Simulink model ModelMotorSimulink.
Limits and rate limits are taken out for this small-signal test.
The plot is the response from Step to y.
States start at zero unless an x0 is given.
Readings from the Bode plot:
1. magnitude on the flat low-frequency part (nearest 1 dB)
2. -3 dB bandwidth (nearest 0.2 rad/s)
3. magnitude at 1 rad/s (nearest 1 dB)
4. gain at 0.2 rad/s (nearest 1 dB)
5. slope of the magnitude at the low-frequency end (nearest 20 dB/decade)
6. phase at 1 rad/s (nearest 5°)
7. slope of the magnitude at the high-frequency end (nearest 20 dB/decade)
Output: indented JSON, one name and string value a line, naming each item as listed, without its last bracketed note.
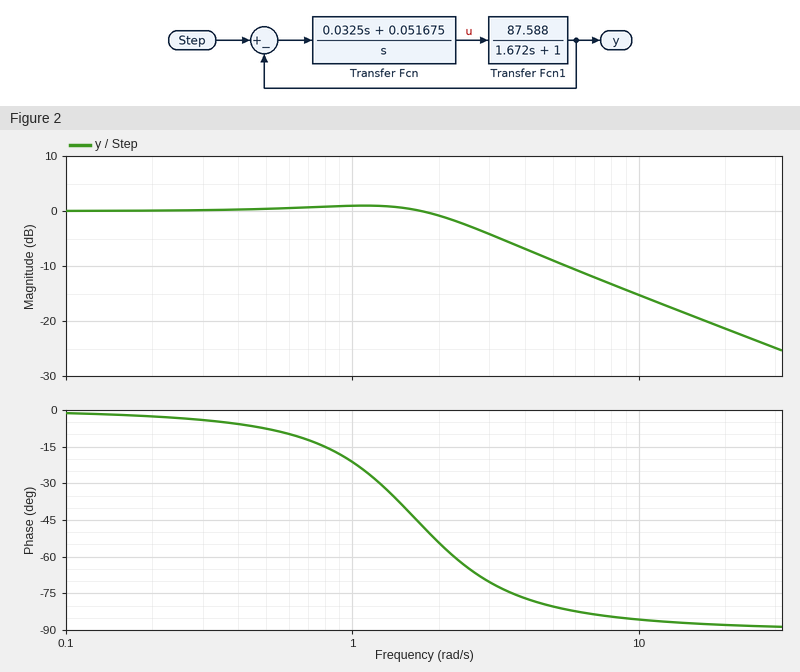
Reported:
{
  "magnitude on the flat low-frequency part": "0 dB",
  "-3 dB bandwidth": "2.6 rad/s",
  "magnitude at 1 rad/s": "1 dB",
  "gain at 0.2 rad/s": "0 dB",
  "slope of the magnitude at the low-frequency end": "0 dB/decade",
  "phase at 1 rad/s": "-20°",
  "slope of the magnitude at the high-frequency end": "-20 dB/decade"
}
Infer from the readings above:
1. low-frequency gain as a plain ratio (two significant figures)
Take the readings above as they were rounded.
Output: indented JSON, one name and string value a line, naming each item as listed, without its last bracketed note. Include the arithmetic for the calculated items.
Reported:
{
  "low-frequency gain as a plain ratio": "10^(0 / 20) = 1.0"
}
